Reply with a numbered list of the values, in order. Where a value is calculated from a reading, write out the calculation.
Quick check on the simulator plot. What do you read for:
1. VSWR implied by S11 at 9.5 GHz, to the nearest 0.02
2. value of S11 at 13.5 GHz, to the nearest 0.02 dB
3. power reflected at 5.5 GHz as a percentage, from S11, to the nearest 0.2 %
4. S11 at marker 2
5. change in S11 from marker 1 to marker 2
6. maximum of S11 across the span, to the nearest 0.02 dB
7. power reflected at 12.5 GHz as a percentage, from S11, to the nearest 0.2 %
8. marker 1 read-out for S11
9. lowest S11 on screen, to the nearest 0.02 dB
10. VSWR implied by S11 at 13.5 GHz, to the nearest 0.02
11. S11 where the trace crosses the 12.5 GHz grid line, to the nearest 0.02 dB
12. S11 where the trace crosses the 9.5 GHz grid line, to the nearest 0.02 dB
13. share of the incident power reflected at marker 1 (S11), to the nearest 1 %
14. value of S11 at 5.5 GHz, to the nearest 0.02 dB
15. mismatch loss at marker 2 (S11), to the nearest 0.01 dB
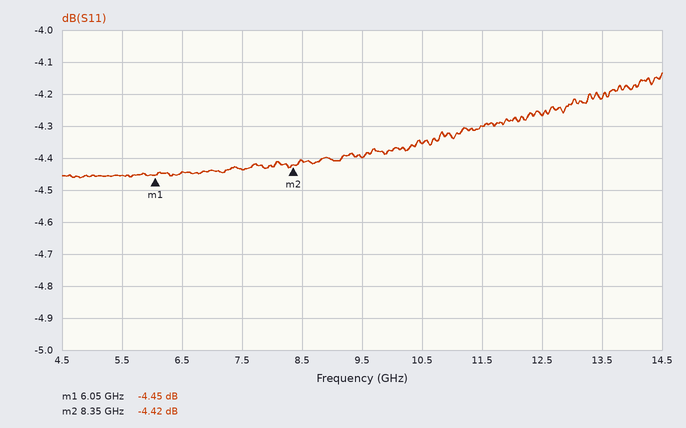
1. |Γ| = 10^(-4.4/20) = 0.6026; VSWR = (1 + 0.6026)/(1 − 0.6026) ≈ 4.03, so 4.04 to the nearest 0.02
2. -4.22 dB
3. 10^(-4.46/10) ≈ 35.8 %
4. -4.42 dB
5. -4.42 − (-4.45) = 0.03 dB
6. -4.14 dB
7. 10^(-4.26/10) ≈ 37.5 %, so 37.4 % to the nearest 0.2 %
8. -4.45 dB
9. -4.46 dB
10. |Γ| = 10^(-4.22/20) = 0.6152; VSWR = (1 + 0.6152)/(1 − 0.6152) ≈ 4.20
11. -4.26 dB
12. -4.40 dB
13. 10^(-4.45/10) ≈ 36 %
14. -4.46 dB
15. −10 log10(1 − 10^(-4.42/10)) ≈ 1.95 dB
